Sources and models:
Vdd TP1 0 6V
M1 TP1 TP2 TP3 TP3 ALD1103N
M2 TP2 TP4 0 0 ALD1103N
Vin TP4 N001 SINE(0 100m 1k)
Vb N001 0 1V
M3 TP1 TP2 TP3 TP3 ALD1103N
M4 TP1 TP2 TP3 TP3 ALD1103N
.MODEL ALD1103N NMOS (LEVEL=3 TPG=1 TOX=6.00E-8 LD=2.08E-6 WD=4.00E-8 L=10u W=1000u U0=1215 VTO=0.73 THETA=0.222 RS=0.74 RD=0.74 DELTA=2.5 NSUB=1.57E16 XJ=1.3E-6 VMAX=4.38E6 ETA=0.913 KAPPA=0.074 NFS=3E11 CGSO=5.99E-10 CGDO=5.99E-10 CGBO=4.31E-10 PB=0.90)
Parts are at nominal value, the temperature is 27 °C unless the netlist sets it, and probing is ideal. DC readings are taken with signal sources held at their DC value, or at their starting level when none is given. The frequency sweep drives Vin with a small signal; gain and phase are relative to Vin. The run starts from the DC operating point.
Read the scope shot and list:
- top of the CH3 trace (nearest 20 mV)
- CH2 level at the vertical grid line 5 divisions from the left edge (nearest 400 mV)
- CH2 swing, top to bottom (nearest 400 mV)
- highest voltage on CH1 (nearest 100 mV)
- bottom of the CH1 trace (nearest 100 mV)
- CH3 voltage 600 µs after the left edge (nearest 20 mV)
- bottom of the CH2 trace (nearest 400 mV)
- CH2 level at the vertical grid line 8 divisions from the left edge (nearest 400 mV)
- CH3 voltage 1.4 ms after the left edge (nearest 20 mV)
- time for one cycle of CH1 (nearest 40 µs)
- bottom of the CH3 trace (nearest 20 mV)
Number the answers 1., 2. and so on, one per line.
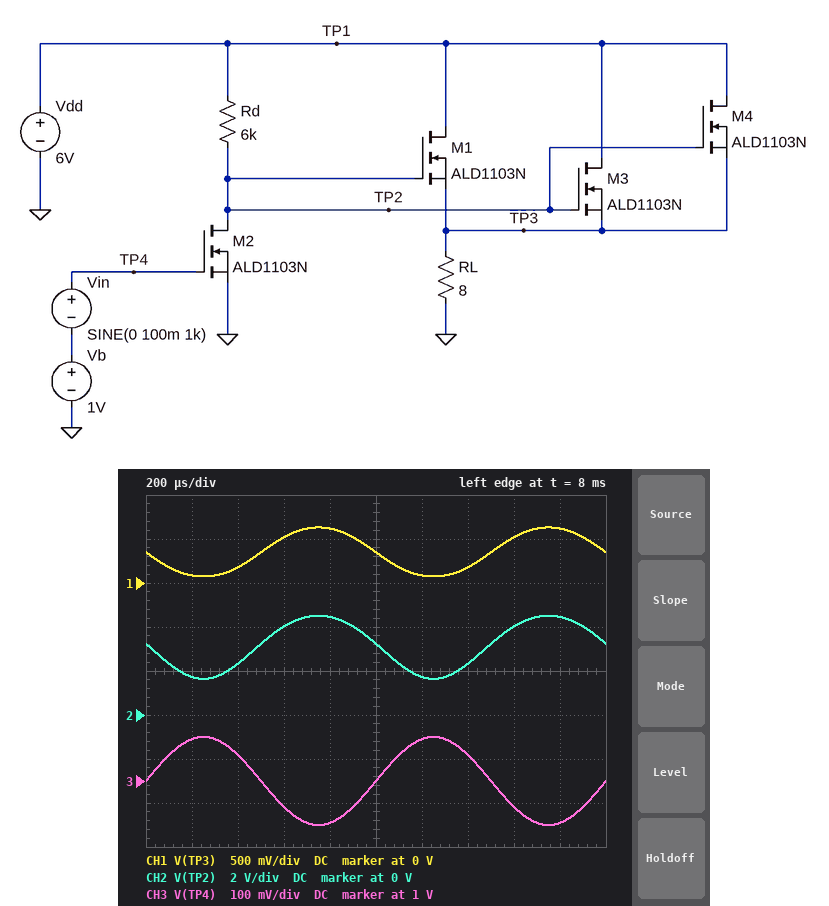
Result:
1. 1.10 V
2. 3.2 V
3. 2.8 V
4. 600 mV
5. 100 mV
6. 940 mV
7. 1.6 V
8. 4.0 V
9. 1.06 V
10. 1.00 ms
11. 900 mV
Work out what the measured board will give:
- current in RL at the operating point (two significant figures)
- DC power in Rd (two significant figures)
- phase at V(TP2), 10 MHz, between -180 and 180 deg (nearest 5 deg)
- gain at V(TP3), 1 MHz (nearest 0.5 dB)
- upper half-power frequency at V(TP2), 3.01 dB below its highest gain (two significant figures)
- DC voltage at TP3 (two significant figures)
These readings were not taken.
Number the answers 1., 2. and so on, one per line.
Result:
1. 44 mA
2. 1.3 mW
3. 105 deg
4. 9.0 dB
5. 3.2 MHz
6. 350 mV
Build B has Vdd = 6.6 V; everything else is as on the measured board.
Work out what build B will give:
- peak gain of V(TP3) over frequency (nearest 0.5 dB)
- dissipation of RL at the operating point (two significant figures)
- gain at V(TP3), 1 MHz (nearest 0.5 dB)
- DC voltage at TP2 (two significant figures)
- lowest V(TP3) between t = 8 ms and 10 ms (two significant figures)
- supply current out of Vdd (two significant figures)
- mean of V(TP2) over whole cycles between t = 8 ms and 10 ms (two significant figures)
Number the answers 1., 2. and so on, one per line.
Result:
1. 10.0 dB
2. 27 mW
3. 9.5 dB
4. 3.8 V
5. 150 mV
6. 59 mA
7. 3.7 V
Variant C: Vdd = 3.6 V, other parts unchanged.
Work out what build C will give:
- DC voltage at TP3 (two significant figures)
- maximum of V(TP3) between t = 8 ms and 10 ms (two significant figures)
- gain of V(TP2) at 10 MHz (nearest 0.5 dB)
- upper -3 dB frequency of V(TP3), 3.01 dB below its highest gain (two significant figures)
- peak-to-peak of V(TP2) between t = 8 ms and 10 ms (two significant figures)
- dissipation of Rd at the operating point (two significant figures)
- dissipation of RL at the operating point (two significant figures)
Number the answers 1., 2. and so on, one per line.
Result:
1. 14 mV
2. 170 mV
3. 11.5 dB
4. 2.8 MHz
5. 2.1 V
6. 1.1 mW
7. 25 µW
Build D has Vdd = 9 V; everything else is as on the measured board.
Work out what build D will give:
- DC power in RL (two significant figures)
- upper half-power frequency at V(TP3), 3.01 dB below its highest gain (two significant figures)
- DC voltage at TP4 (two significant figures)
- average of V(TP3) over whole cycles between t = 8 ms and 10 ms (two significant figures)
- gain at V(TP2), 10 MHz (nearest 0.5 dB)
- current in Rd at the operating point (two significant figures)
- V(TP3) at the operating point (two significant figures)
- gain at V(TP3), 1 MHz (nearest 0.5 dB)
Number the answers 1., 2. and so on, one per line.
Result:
1. 120 mW
2. 3.4 MHz
3. 1.0 V
4. 980 mV
5. 13.5 dB
6. 510 µA
7. 990 mV
8. 11.5 dB
